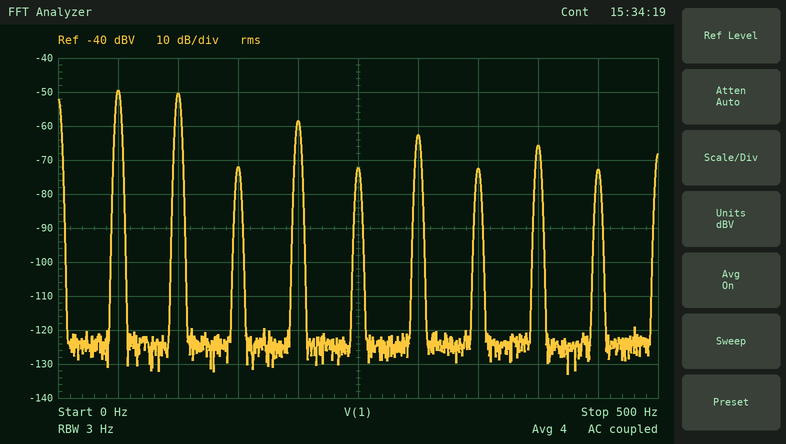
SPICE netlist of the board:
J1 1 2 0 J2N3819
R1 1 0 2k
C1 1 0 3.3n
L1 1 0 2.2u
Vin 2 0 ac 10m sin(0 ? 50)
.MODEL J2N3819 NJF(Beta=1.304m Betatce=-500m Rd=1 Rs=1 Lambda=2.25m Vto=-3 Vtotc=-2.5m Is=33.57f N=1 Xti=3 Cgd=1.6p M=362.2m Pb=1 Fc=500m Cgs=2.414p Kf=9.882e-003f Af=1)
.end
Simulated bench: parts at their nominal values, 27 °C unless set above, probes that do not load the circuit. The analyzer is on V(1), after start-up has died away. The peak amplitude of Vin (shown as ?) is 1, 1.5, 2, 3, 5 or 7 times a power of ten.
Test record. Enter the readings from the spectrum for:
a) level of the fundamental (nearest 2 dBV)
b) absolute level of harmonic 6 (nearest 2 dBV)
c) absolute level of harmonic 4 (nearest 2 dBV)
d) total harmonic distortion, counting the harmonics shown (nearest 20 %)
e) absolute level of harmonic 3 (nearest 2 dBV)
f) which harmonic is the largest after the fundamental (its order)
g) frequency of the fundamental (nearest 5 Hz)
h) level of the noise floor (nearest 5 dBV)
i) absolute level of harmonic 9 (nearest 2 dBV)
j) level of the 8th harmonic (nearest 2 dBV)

-50 dBV
-62 dBV
-58 dBV
100 %
-72 dBV
2
50 Hz
-125 dBV
-72 dBV
-66 dBV
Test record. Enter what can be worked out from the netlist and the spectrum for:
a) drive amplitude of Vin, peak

15 V
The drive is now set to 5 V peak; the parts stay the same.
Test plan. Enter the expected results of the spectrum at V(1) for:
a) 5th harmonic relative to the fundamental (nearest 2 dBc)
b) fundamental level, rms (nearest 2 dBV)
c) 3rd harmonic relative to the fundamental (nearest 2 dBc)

-14 dBc
-60 dBV
-12 dBc
